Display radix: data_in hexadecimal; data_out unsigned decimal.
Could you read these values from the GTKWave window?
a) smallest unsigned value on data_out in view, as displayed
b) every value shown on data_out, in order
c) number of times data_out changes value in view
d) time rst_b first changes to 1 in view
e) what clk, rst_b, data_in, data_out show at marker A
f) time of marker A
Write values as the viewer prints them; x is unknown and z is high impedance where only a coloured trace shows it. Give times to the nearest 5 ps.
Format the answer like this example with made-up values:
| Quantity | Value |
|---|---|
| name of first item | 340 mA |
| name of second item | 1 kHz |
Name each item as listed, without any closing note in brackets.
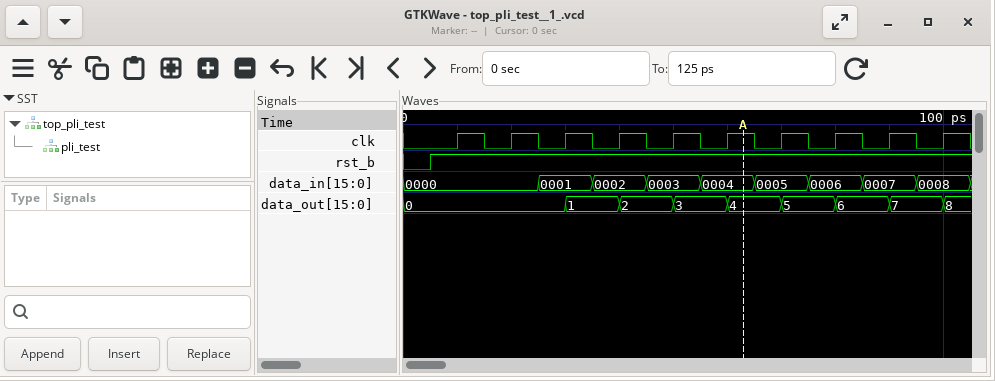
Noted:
| Quantity | Value |
|---|---|
| smallest unsigned value on data_out in view, as displayed | 0 |
| every value shown on data_out, in order | 0, 1, 2, 3, 4, 5, 6, 7, 8 |
| number of times data_out changes value in view | 8 |
| time rst_b first changes to 1 in view | 5 ps |
| what clk, rst_b, data_in, data_out show at marker A | clk=1, rst_b=1, data_in=0004, data_out=4 |
| time of marker A | 65 ps |
